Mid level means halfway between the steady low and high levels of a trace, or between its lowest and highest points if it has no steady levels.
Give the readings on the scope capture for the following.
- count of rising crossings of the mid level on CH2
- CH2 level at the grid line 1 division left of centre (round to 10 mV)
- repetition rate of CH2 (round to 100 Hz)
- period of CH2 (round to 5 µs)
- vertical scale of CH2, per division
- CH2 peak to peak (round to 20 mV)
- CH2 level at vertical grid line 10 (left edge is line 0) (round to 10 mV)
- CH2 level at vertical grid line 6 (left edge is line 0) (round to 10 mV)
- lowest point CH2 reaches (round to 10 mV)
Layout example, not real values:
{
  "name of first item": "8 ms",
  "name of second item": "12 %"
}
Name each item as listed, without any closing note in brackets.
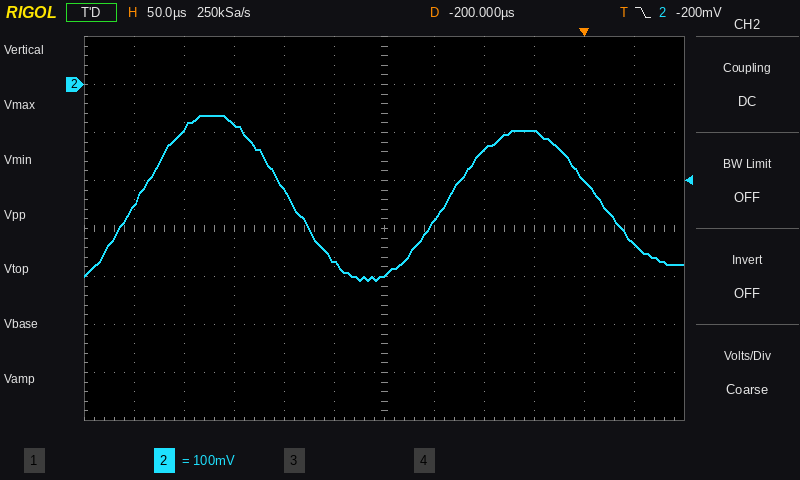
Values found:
{
  "count of rising crossings of the mid level on CH2": "2",
  "CH2 level at the grid line 1 division left of centre": "-370 mV",
  "repetition rate of CH2": "3.2 kHz",
  "period of CH2": "310 µs",
  "vertical scale of CH2, per division": "100 mV",
  "CH2 peak to peak": "340 mV",
  "CH2 level at vertical grid line 10 (left edge is line 0)": "-200 mV",
  "CH2 level at vertical grid line 6 (left edge is line 0)": "-400 mV",
  "lowest point CH2 reaches": "-410 mV"
}
